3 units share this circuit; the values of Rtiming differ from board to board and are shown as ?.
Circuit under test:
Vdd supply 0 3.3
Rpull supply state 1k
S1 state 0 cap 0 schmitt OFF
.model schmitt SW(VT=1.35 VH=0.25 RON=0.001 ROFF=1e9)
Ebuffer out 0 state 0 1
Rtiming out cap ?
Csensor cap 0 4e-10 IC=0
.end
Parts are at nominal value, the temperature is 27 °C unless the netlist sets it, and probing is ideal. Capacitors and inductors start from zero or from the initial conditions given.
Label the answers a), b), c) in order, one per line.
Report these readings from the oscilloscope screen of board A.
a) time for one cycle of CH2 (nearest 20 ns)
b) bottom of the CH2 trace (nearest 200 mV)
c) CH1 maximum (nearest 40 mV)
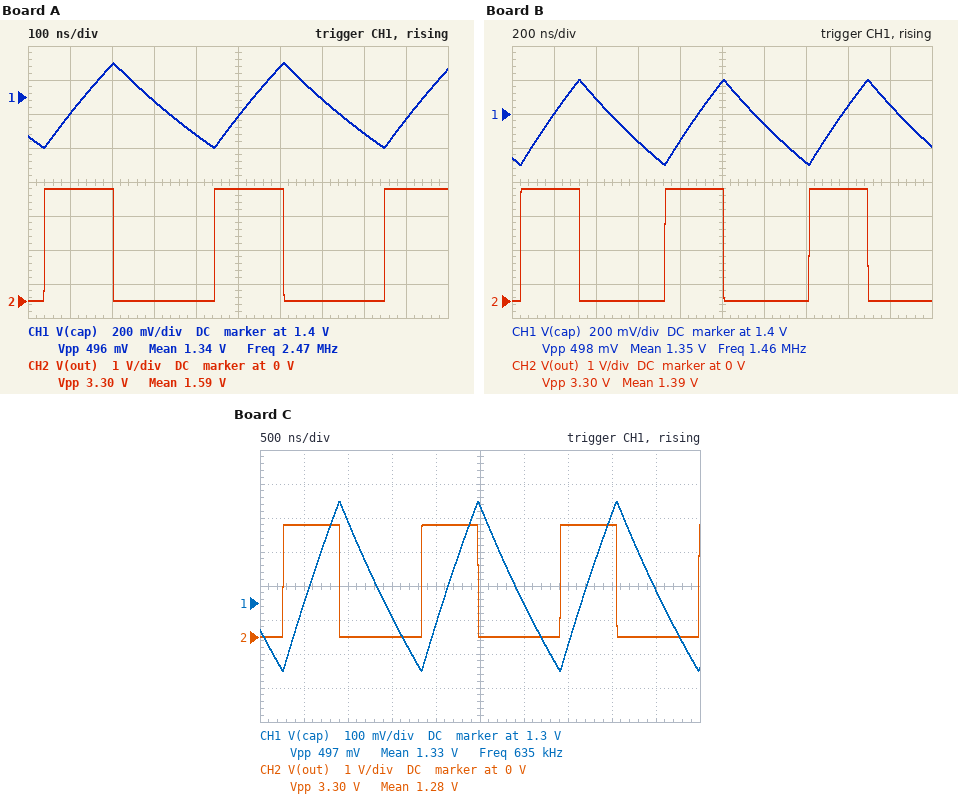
a) 400 ns
b) 0 V
c) 1.60 V
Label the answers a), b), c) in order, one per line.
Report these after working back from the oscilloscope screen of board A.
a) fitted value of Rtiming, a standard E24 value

a) 1.6 kΩ
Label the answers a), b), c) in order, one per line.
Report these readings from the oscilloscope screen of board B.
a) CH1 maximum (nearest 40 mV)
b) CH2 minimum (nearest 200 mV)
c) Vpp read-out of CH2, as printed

a) 1.60 V
b) 0 V
c) 3.30 V
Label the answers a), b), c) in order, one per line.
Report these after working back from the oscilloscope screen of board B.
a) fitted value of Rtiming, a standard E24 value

a) 2.7 kΩ
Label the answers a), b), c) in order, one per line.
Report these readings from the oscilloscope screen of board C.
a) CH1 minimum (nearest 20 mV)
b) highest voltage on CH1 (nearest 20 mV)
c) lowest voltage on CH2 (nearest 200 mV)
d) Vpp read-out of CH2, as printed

a) 1.10 V
b) 1.60 V
c) 0 V
d) 3.30 V
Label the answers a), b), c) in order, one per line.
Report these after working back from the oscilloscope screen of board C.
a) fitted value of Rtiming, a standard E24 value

a) 6.2 kΩ
